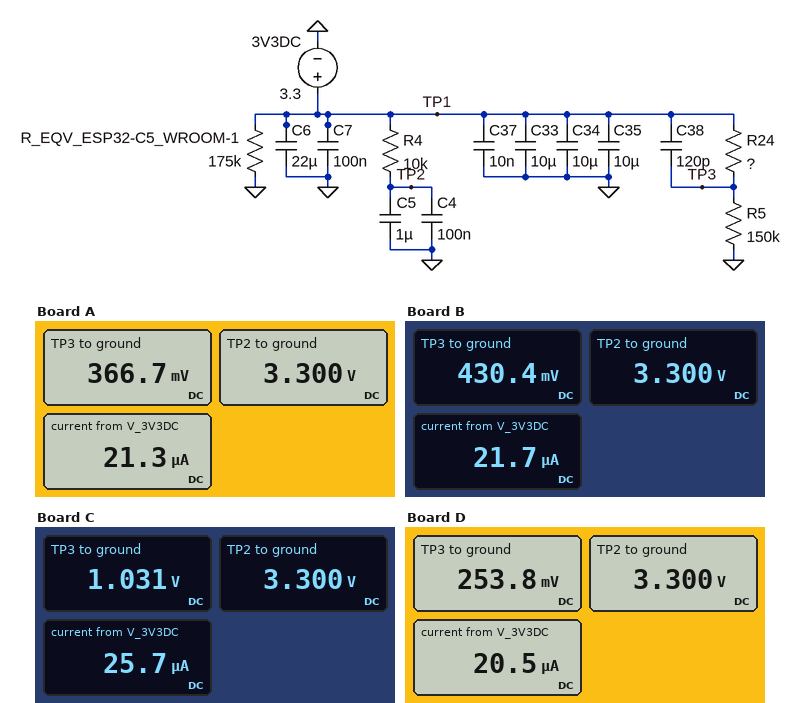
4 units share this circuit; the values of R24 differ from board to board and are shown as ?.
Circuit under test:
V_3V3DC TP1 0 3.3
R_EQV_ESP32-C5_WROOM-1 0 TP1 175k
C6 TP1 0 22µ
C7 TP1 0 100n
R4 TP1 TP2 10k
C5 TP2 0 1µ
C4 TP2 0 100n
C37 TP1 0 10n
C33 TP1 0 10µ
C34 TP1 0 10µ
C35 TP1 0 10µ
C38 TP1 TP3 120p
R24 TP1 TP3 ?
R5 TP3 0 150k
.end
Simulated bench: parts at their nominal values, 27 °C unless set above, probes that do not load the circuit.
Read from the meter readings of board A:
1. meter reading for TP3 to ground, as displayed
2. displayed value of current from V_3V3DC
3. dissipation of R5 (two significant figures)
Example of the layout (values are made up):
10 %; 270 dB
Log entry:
366.7 mV; 21.3 µA; 900 nW
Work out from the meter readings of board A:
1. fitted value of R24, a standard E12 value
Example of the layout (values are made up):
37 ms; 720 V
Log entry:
1.2 MΩ
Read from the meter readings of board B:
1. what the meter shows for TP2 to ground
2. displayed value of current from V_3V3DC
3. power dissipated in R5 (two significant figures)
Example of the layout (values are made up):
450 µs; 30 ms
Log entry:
3.300 V; 21.7 µA; 1.2 µW
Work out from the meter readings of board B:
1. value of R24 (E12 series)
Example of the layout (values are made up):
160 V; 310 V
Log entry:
1 MΩ
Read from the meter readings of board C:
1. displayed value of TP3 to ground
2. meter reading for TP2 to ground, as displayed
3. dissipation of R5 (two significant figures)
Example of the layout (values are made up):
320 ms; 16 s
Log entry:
1.031 V; 3.300 V; 7.1 µW
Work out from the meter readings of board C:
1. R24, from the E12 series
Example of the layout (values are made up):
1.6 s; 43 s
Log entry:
330 kΩ
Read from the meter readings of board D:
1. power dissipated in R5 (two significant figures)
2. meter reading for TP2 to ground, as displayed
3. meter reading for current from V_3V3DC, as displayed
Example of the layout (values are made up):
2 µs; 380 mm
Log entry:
430 nW; 3.300 V; 20.5 µA
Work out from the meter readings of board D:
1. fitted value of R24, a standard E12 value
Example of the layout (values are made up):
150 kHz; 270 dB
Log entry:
1.8 MΩ
